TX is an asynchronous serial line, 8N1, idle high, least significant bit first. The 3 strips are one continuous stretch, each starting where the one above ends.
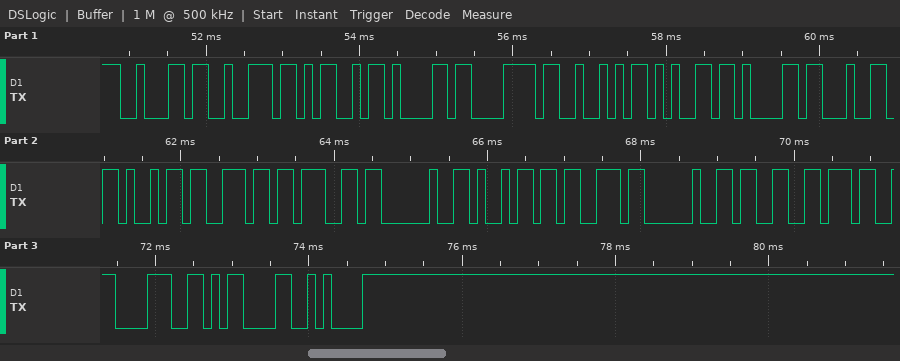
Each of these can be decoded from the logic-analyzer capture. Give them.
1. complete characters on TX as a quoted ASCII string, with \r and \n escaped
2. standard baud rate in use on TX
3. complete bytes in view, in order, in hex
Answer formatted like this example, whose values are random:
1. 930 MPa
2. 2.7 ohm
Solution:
1. "brMaxReading is 378\r\n"
2. 9600 baud
3. 62 72 4D 61 78 52 65 61 64 69 6E 67 20 69 73 20 33 37 38 0D 0A
